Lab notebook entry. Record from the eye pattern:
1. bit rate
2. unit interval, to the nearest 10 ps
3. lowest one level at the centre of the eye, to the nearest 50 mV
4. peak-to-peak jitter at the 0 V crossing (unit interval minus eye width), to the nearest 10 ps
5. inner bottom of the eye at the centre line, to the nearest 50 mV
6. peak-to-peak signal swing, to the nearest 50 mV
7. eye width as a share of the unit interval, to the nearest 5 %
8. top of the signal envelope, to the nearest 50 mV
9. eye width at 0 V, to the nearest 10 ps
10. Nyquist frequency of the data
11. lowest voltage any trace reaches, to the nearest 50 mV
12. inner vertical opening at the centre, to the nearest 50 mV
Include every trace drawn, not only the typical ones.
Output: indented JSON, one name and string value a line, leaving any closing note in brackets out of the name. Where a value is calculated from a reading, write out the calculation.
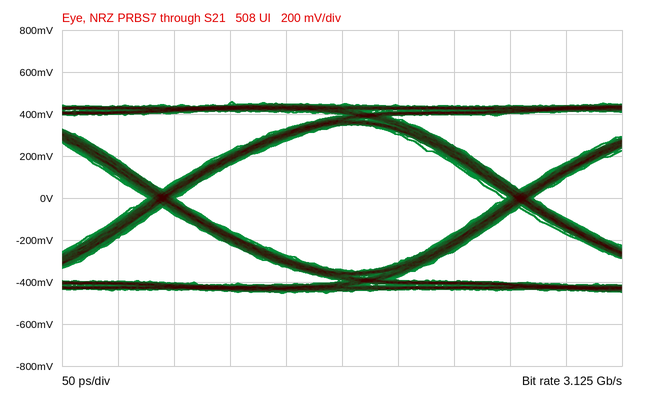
{
  "bit rate": "3.125 Gb/s",
  "unit interval, to the nearest 10 ps": "320 ps",
  "lowest one level at the centre of the eye, to the nearest 50 mV": "350 mV",
  "peak-to-peak jitter at the 0 V crossing (unit interval minus eye width), to the nearest 10 ps": "30 ps",
  "inner bottom of the eye at the centre line, to the nearest 50 mV": "-350 mV",
  "peak-to-peak signal swing, to the nearest 50 mV": "900 mV",
  "eye width as a share of the unit interval, to the nearest 5 %": "290 ps / 320 ps ≈ 90.6 %, so 90 % to the nearest 5 %",
  "top of the signal envelope, to the nearest 50 mV": "450 mV",
  "eye width at 0 V, to the nearest 10 ps": "290 ps",
  "Nyquist frequency of the data": "1.5625 GHz",
  "lowest voltage any trace reaches, to the nearest 50 mV": "-450 mV",
  "inner vertical opening at the centre, to the nearest 50 mV": "700 mV"
}
